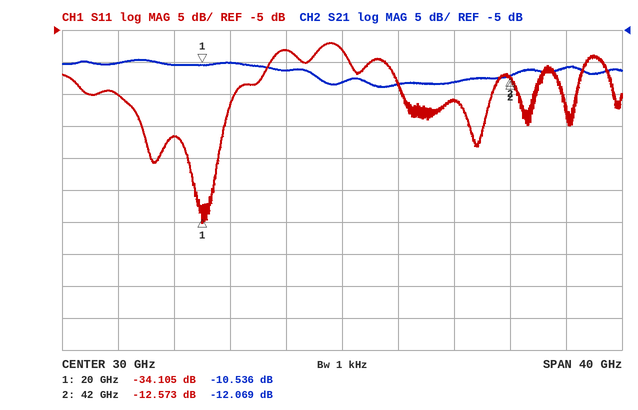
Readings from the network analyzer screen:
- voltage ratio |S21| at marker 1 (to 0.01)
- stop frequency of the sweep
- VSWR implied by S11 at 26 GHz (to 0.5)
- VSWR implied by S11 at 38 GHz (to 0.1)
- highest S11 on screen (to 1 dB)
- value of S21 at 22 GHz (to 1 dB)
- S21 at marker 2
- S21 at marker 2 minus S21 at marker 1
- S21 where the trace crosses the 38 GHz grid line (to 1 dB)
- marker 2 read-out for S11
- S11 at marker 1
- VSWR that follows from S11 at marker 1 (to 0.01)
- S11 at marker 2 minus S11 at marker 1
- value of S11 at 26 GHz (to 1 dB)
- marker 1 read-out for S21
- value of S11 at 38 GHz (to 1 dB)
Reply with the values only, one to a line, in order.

0.30
50 GHz
2.5
1.4
-7 dB
-10 dB
-12.069 dB
-1.533 dB
-13 dB
-12.573 dB
-34.105 dB
1.04
21.532 dB
-8 dB
-10.536 dB
-16 dB
